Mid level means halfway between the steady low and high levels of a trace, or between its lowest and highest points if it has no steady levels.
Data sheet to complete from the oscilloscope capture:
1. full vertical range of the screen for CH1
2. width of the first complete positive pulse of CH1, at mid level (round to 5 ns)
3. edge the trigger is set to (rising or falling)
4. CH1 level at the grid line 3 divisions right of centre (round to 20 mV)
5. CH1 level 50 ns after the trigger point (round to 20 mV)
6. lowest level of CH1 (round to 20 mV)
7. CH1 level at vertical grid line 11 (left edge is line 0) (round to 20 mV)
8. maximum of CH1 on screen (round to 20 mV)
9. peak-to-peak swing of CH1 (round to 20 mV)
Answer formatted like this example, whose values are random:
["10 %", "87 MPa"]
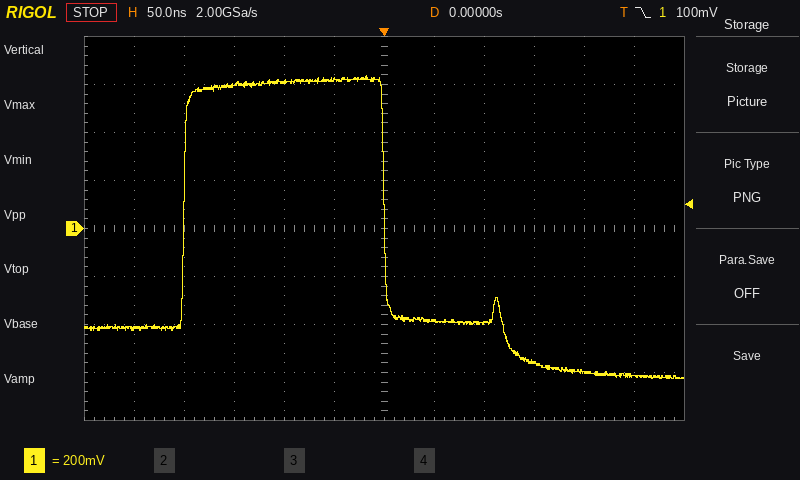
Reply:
["1.6 V", "200 ns", "falling", "-560 mV", "-380 mV", "-620 mV", "-620 mV", "640 mV", "1.26 V"]
